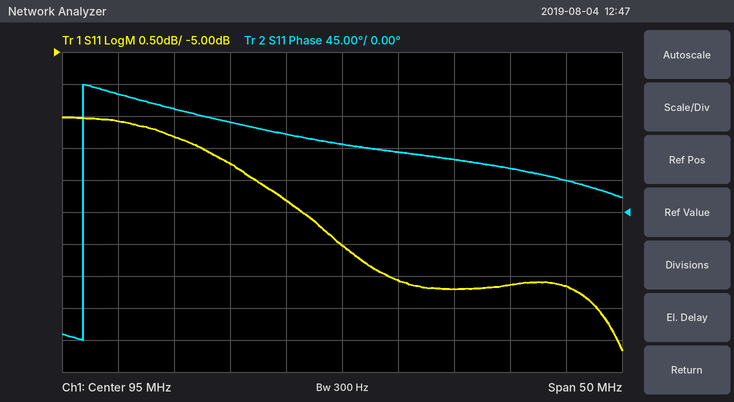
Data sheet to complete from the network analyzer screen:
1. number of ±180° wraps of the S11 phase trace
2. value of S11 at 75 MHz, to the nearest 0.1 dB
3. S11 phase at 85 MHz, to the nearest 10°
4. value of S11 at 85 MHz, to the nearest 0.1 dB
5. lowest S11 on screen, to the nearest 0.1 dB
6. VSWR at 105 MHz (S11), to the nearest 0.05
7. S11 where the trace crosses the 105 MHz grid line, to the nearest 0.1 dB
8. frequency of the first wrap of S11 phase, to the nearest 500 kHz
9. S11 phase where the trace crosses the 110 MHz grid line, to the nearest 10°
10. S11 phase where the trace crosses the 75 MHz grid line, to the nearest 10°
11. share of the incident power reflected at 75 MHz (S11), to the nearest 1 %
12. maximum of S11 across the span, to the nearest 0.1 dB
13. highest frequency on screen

1
-6.1 dB
130°
-6.7 dB
-9.7 dB
2.15
-8.7 dB
72.0 MHz
60°
170°
25 %
-6.0 dB
120 MHz
